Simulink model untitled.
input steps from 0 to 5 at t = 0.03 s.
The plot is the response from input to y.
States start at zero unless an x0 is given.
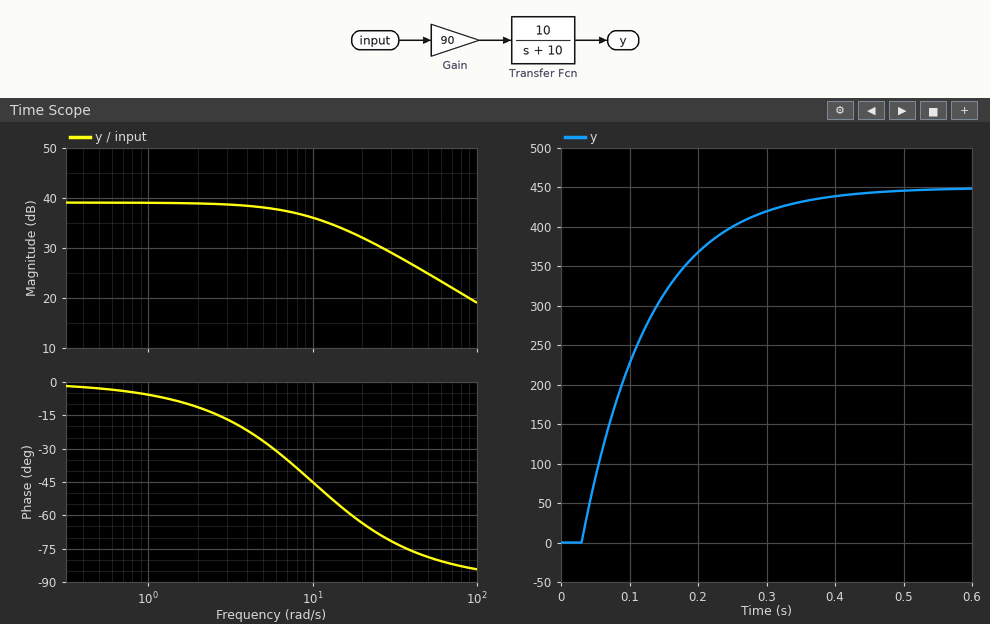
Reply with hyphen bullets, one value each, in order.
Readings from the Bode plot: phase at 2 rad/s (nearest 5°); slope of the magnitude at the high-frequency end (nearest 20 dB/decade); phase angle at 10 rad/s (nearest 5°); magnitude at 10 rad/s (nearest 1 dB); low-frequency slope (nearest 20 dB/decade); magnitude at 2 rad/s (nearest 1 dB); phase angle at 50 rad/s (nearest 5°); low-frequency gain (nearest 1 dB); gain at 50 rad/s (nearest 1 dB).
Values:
- -10°
- -20 dB/decade
- -45°
- 36 dB
- 0 dB/decade
- 39 dB
- -80°
- 39 dB
- 25 dB
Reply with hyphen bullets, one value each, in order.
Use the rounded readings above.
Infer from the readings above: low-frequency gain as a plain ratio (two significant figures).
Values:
- 89
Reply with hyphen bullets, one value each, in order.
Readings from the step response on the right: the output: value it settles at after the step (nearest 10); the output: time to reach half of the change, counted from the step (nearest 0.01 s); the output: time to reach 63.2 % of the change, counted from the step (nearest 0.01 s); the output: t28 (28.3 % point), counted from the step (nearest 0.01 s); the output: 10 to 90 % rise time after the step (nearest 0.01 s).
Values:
- 450
- 0.07 s
- 0.10 s
- 0.03 s
- 0.22 s
